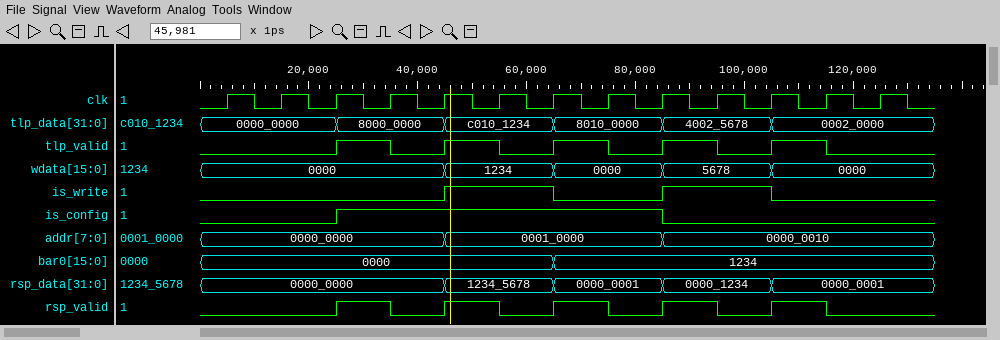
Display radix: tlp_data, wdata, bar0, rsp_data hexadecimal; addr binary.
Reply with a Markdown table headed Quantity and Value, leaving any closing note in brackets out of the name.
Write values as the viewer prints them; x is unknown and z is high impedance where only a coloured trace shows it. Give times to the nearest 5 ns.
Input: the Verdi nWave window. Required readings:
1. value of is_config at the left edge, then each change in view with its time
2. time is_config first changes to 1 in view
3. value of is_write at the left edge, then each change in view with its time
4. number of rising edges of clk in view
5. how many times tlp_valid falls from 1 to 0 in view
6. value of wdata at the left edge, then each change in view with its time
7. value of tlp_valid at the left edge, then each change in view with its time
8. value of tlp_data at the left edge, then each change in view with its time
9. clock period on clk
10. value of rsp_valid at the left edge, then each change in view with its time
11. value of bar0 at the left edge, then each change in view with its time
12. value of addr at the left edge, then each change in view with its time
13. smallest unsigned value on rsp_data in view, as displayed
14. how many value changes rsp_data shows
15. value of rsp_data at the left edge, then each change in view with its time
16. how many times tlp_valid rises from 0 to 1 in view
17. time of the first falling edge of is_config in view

| Quantity | Value |
|---|---|
| value of is_config at the left edge, then each change in view with its time | 0, 1 at 25 ns, 0 at 85 ns |
| time is_config first changes to 1 in view | 25 ns |
| value of is_write at the left edge, then each change in view with its time | 0, 1 at 45 ns, 0 at 65 ns, 1 at 85 ns, 0 at 105 ns |
| number of rising edges of clk in view | 13 |
| how many times tlp_valid falls from 1 to 0 in view | 5 |
| value of wdata at the left edge, then each change in view with its time | 0000, 1234 at 45 ns, 0000 at 65 ns, 5678 at 85 ns, 0000 at 105 ns |
| value of tlp_valid at the left edge, then each change in view with its time | 0, 1 at 25 ns, 0 at 35 ns, 1 at 45 ns, 0 at 55 ns, 1 at 65 ns, 0 at 75 ns, 1 at 85 ns, 0 at 95 ns, 1 at 105 ns, 0 at 115 ns |
| value of tlp_data at the left edge, then each change in view with its time | 0000_0000, 8000_0000 at 25 ns, c010_1234 at 45 ns, 8010_0000 at 65 ns, 4002_5678 at 85 ns, 0002_0000 at 105 ns |
| clock period on clk | 10 ns |
| value of rsp_valid at the left edge, then each change in view with its time | 0, 1 at 25 ns, 0 at 35 ns, 1 at 45 ns, 0 at 55 ns, 1 at 65 ns, 0 at 75 ns, 1 at 85 ns, 0 at 95 ns, 1 at 105 ns, 0 at 115 ns |
| value of bar0 at the left edge, then each change in view with its time | 0000, 1234 at 65 ns |
| value of addr at the left edge, then each change in view with its time | 0000_0000, 0001_0000 at 45 ns, 0000_0010 at 85 ns |
| smallest unsigned value on rsp_data in view, as displayed | 0000_0000 |
| how many value changes rsp_data shows | 4 |
| value of rsp_data at the left edge, then each change in view with its time | 0000_0000, 1234_5678 at 45 ns, 0000_0001 at 65 ns, 0000_1234 at 85 ns, 0000_0001 at 105 ns |
| how many times tlp_valid rises from 0 to 1 in view | 5 |
| time of the first falling edge of is_config in view | 85 ns |
